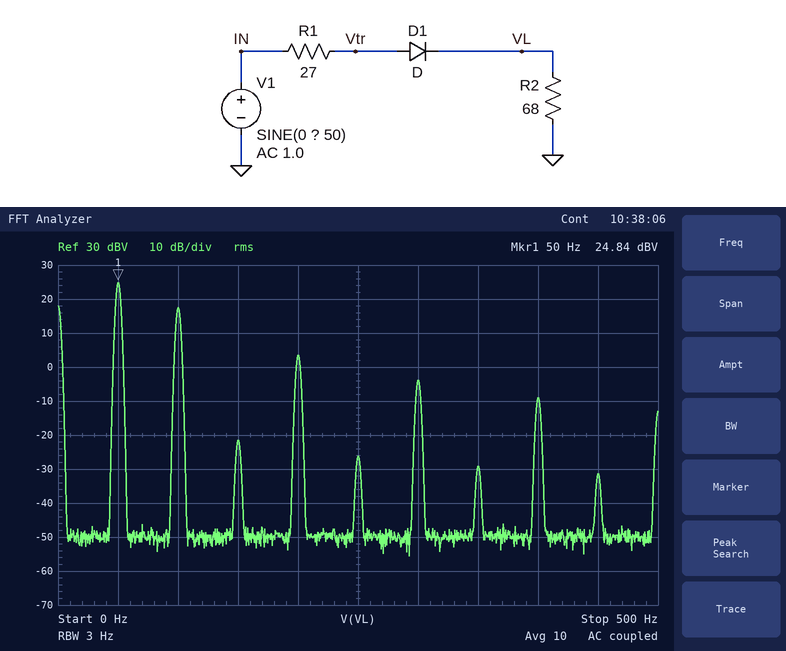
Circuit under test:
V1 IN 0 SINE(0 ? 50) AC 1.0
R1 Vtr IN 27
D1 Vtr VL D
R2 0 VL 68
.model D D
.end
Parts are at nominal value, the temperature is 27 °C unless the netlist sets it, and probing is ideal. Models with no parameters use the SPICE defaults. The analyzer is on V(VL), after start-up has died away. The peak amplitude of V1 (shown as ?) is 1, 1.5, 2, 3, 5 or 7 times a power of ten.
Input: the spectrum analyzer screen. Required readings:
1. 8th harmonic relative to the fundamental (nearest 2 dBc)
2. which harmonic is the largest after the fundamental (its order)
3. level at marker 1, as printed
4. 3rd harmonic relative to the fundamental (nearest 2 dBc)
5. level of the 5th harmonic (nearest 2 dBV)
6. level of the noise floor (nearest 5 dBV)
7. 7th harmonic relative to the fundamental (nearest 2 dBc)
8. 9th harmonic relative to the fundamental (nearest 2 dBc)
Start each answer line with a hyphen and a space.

- -34 dBc
- 2
- 24.84 dBV
- -46 dBc
- -26 dBV
- -50 dBV
- -54 dBc
- -56 dBc
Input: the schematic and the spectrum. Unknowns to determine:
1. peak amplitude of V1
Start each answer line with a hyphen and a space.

- 70 V
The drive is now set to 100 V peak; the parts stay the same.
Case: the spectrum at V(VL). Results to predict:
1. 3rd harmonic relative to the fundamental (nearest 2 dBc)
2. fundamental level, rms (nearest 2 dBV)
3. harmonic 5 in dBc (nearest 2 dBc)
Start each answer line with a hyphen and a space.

- -50 dBc
- 28 dBV
- -54 dBc
